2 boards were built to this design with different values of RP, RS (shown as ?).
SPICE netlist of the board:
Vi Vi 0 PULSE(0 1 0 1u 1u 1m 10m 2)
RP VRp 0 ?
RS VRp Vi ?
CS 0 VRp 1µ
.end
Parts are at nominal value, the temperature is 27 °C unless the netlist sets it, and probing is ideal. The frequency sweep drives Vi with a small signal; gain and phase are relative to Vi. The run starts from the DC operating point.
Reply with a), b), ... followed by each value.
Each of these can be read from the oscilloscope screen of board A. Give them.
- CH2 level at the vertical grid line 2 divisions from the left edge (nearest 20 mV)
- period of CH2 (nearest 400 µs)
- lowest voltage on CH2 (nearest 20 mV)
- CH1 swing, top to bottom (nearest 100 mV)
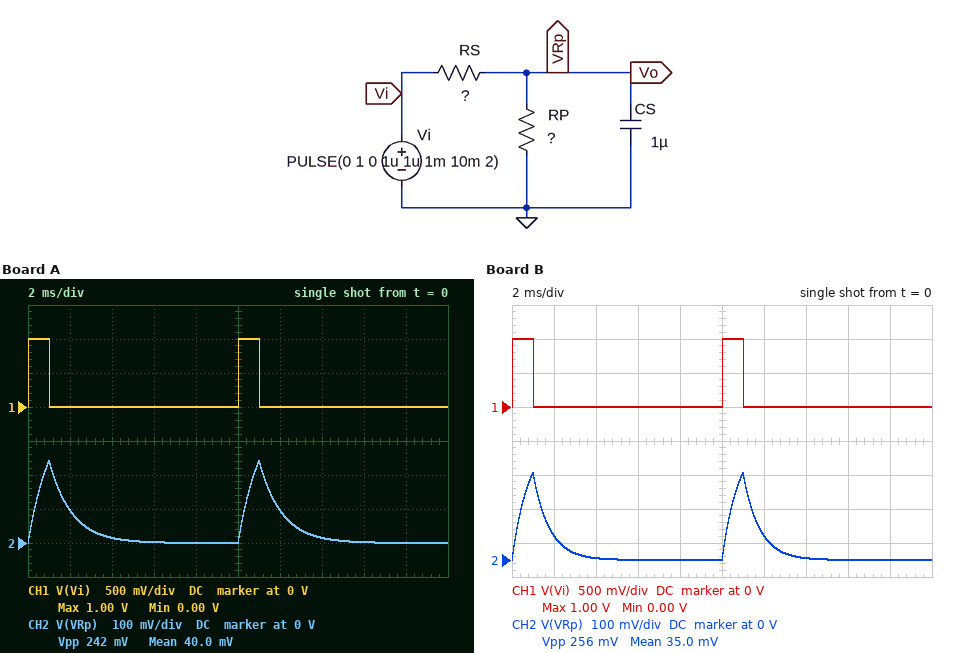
a) 20 mV
b) 10.0 ms
c) 0 V
d) 1.0 V
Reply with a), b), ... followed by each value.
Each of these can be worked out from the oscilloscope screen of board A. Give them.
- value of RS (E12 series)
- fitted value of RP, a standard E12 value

a) 2.7 kΩ
b) 1.8 kΩ
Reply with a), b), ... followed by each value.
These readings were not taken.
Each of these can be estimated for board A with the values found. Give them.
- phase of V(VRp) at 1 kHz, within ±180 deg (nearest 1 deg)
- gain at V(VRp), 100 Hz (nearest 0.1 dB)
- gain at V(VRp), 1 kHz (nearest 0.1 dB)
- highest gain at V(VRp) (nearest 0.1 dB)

a) -82 deg
b) -9.6 dB
c) -24.7 dB
d) -8.0 dB
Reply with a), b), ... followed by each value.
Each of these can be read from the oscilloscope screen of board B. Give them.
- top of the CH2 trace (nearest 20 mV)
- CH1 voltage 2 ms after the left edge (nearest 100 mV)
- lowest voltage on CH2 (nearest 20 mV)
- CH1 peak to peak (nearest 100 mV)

a) 260 mV
b) 0 V
c) 0 V
d) 1.0 V
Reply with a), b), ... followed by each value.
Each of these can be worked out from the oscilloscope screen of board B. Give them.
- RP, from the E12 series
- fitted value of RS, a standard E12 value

a) 1.2 kΩ
b) 2.2 kΩ
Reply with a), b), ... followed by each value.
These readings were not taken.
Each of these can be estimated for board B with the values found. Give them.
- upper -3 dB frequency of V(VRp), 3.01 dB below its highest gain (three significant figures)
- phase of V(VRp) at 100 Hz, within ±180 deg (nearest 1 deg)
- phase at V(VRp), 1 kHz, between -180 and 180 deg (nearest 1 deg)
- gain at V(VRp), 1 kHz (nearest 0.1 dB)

a) 205 Hz
b) -26 deg
c) -78 deg
d) -23.0 dB
